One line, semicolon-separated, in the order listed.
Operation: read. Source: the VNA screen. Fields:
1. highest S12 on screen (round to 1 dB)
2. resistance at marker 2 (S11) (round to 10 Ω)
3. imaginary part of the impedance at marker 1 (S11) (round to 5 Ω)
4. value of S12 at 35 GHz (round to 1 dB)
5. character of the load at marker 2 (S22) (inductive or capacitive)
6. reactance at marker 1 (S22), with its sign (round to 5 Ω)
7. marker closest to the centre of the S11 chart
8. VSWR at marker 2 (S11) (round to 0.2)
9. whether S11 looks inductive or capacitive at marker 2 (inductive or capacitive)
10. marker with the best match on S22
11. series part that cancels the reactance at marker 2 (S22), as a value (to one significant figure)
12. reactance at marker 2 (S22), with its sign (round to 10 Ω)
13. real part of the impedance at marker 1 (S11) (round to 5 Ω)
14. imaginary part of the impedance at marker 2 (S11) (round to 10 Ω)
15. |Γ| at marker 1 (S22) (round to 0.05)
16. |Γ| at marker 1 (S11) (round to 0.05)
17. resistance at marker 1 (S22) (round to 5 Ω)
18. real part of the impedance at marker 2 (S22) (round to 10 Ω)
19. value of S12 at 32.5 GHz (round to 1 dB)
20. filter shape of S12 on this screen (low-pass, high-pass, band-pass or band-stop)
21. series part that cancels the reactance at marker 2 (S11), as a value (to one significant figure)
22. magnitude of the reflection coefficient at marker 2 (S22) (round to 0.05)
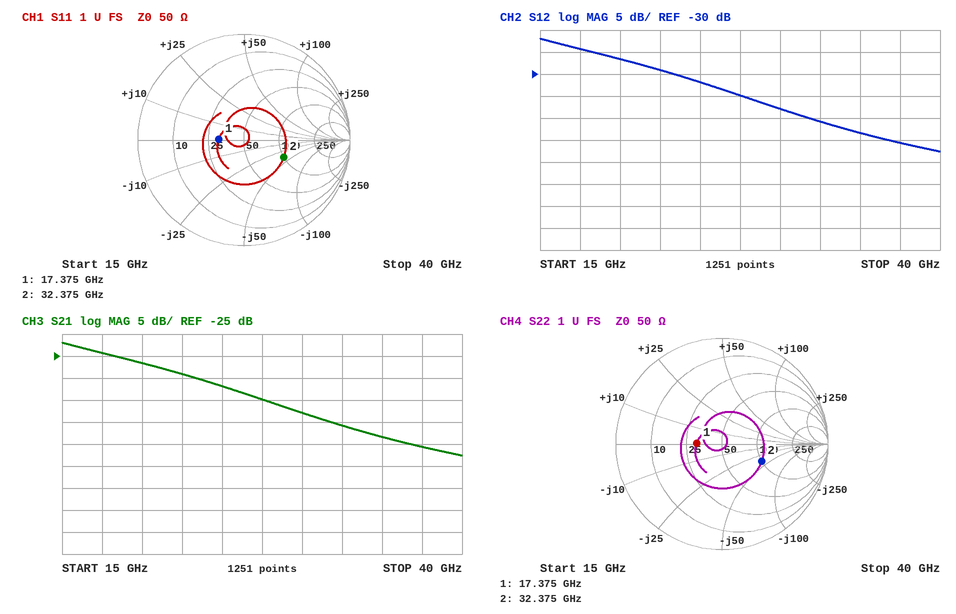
-22 dB; 100 Ω; 0 Ω; -43 dB; capacitive; 0 Ω; marker 1; 2.4; capacitive; marker 1; 200 pH; -40 Ω; 30 Ω; -40 Ω; 0.25; 0.25; 30 Ω; 100 Ω; -41 dB; low-pass; 200 pH; 0.40
